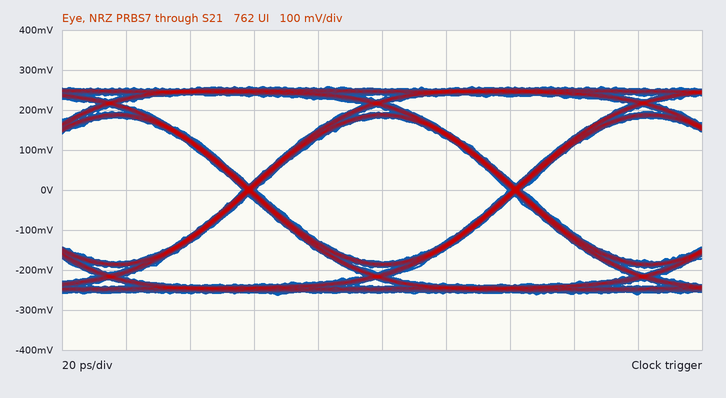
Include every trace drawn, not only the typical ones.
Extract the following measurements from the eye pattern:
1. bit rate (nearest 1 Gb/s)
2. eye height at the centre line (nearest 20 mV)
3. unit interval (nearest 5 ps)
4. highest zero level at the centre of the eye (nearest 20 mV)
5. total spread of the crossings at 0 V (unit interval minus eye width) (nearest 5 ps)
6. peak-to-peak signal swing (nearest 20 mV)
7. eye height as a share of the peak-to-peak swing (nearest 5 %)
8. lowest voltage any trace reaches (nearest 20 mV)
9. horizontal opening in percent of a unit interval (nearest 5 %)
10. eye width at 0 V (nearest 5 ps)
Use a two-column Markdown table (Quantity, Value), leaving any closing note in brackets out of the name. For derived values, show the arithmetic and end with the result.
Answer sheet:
| Quantity | Value |
|---|---|
| bit rate | 12 Gb/s |
| eye height at the centre line | 360 mV |
| unit interval | 85 ps |
| highest zero level at the centre of the eye | -180 mV |
| total spread of the crossings at 0 V (unit interval minus eye width) | 5 ps |
| peak-to-peak signal swing | 520 mV |
| eye height as a share of the peak-to-peak swing | 360 mV / 520 mV ≈ 69.2 %, so 70 % to the nearest 5 % |
| lowest voltage any trace reaches | -260 mV |
| horizontal opening in percent of a unit interval | 80 ps / 85 ps ≈ 94.1 %, so 95 % to the nearest 5 % |
| eye width at 0 V | 80 ps |
